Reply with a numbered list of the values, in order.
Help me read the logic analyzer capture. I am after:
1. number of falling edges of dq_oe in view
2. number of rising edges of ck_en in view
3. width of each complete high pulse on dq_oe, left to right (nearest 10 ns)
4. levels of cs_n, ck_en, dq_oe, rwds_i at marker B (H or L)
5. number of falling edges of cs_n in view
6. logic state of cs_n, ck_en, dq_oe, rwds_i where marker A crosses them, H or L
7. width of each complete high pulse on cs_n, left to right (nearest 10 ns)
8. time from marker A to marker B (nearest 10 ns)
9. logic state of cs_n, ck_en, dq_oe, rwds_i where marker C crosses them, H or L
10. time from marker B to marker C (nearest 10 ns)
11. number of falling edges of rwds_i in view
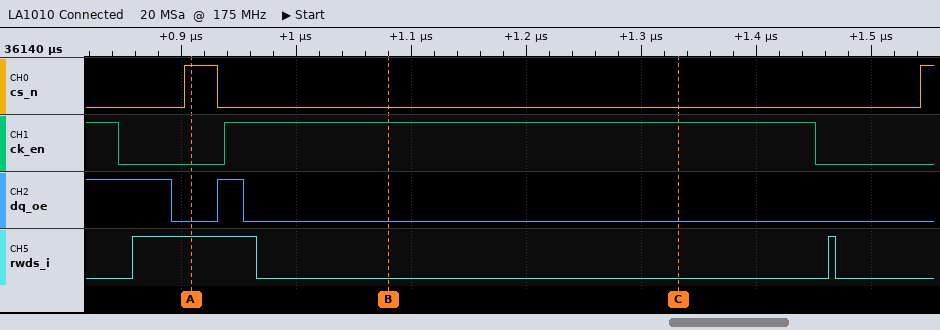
1. 2
2. 1
3. 20 ns
4. cs_n=L, ck_en=H, dq_oe=L, rwds_i=L
5. 1
6. cs_n=H, ck_en=L, dq_oe=L, rwds_i=H
7. 30 ns
8. 170 ns
9. cs_n=L, ck_en=H, dq_oe=L, rwds_i=L
10. 250 ns
11. 2
